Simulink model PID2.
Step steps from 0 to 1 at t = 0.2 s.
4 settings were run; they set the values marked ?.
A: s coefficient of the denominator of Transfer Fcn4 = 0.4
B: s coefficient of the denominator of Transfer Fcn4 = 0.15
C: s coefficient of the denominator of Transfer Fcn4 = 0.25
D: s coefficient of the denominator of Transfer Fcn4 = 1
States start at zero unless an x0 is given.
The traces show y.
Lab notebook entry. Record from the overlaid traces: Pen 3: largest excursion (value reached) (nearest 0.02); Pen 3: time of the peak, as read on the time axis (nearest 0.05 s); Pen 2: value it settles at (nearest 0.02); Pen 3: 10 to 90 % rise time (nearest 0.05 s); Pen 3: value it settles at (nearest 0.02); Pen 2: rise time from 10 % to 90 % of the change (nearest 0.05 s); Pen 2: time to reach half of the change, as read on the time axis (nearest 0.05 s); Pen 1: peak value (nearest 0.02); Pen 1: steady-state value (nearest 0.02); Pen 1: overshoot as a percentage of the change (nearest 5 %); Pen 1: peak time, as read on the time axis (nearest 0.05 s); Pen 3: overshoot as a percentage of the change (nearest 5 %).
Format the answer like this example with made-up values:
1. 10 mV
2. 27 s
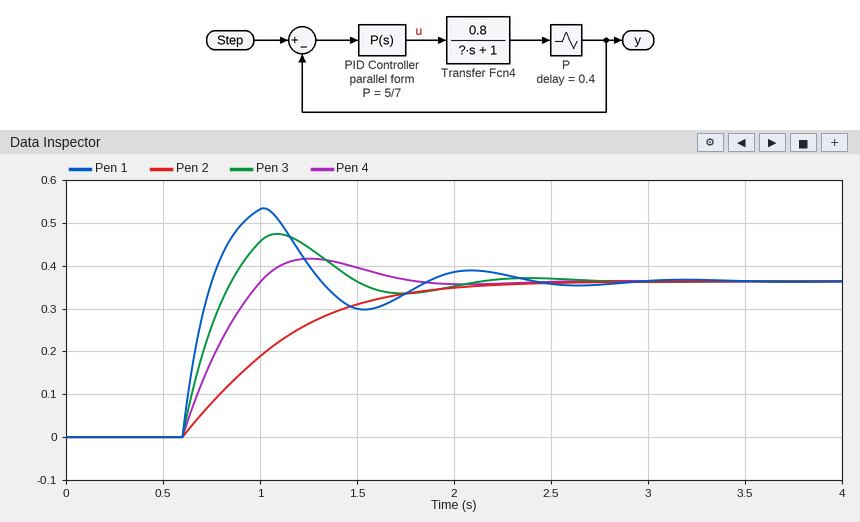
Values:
1. 0.48
2. 1.10 s
3. 0.36
4. 0.20 s
5. 0.36
6. 1.00 s
7. 1.00 s
8. 0.54
9. 0.36
10. 45 %
11. 1.00 s
12. 30 %
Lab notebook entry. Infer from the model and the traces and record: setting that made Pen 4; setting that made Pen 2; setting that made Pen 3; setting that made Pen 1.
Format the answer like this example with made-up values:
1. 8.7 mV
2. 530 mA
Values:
1. A
2. D
3. C
4. B
